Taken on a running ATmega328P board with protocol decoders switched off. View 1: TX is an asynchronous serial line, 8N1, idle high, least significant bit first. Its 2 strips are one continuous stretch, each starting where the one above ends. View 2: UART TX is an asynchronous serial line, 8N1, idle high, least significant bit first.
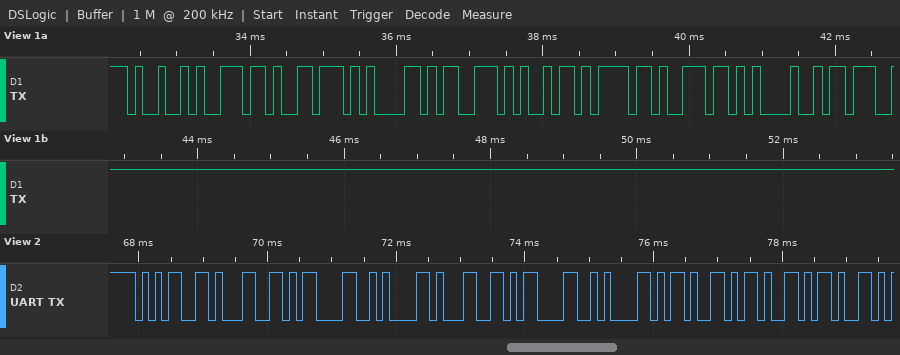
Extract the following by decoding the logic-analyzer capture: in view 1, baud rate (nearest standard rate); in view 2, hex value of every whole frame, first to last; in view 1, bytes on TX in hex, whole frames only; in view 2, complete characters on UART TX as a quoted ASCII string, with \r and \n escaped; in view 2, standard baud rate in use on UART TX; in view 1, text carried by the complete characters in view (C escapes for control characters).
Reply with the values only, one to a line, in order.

9600 baud
35 31 0D 0A 31 0D 0A 2D 2D 2D
0x49 0x6E 0x76 0x61 0x73 0x69 0x6F 0x6E 0x21 0x3B
"51\r\n1\r\n---"
9600 baud
"Invasion!;"
